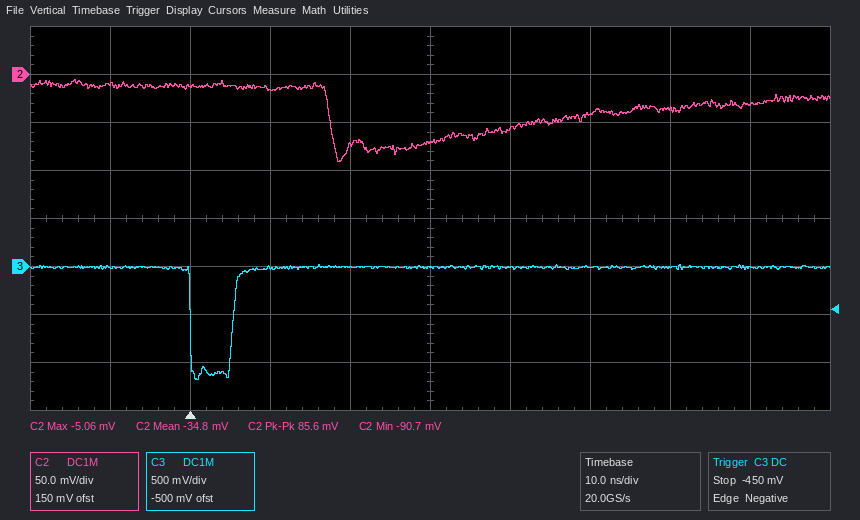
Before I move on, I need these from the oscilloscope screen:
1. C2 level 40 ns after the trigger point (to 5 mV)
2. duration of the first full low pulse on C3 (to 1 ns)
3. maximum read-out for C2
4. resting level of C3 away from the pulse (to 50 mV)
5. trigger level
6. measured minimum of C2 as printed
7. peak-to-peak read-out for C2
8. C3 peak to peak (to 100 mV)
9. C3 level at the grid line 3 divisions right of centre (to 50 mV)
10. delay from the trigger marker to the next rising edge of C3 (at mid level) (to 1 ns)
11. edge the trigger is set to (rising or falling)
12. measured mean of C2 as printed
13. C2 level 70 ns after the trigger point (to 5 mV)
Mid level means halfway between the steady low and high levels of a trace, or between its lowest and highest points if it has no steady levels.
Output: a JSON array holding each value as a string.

["-55 mV", "5 ns", "-5.06 mV", "0 mV", "-450 mV", "-90.7 mV", "85.6 mV", "1.20 V", "0 mV", "5 ns", "falling", "-34.8 mV", "-30 mV"]
